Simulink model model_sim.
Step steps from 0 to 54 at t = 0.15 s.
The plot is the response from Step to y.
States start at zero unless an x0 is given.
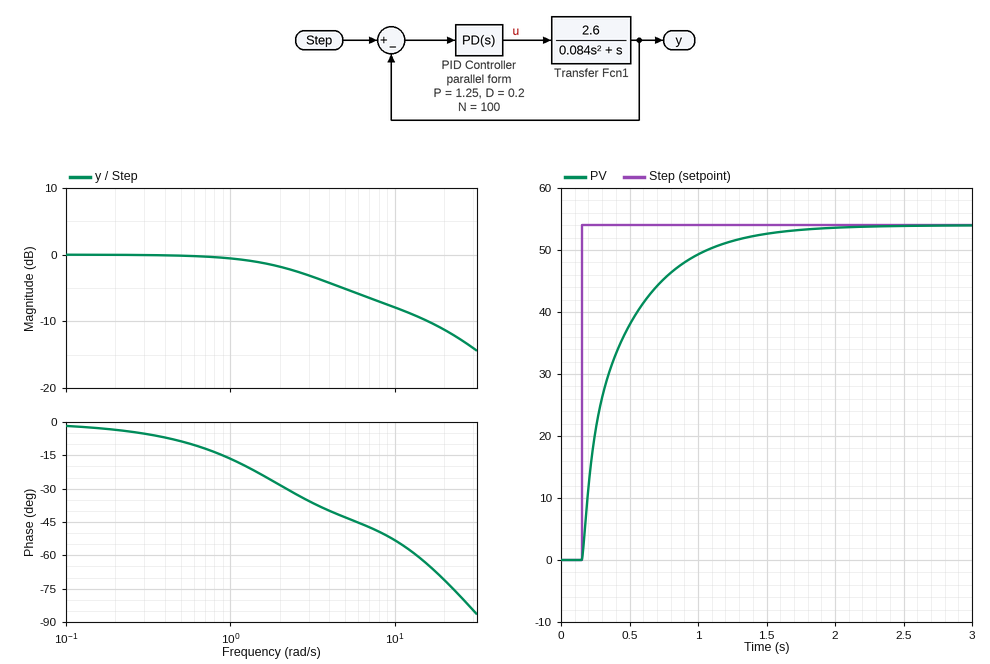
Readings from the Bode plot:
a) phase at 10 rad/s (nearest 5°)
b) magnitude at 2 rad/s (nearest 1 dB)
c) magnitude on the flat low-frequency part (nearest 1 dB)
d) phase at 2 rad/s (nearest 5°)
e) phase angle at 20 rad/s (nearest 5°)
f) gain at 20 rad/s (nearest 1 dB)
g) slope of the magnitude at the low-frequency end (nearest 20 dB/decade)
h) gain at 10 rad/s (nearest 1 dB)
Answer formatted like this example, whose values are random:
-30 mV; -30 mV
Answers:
-55°; -2 dB; 0 dB; -30°; -70°; -11 dB; 0 dB/decade; -8 dB
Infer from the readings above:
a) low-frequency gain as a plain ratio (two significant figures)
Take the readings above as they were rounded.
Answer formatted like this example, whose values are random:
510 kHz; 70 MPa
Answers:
1.0
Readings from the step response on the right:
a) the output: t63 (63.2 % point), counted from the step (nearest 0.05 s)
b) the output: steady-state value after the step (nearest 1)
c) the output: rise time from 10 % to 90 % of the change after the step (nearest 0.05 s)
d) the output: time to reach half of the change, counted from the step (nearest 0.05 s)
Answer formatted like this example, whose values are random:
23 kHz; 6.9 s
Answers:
0.25 s; 54; 0.75 s; 0.15 s
